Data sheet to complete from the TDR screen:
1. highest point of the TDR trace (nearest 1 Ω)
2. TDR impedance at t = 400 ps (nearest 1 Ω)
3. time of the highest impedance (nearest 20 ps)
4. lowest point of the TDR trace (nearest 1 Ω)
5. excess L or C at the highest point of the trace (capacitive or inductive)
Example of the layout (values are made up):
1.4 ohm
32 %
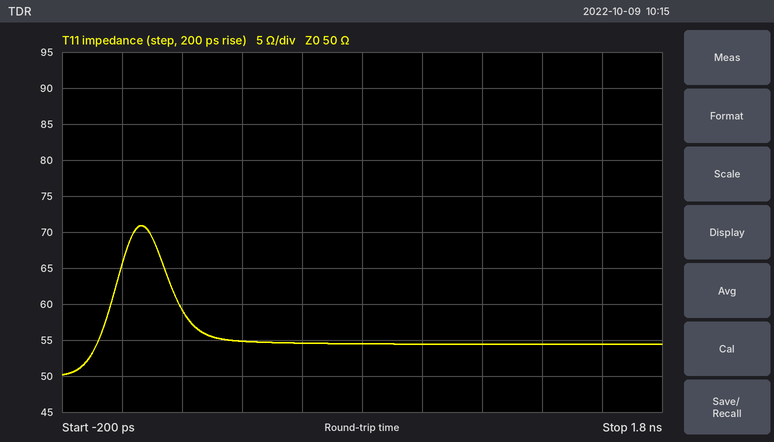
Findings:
71 Ω
55 Ω
60 ps
50 Ω
inductive
